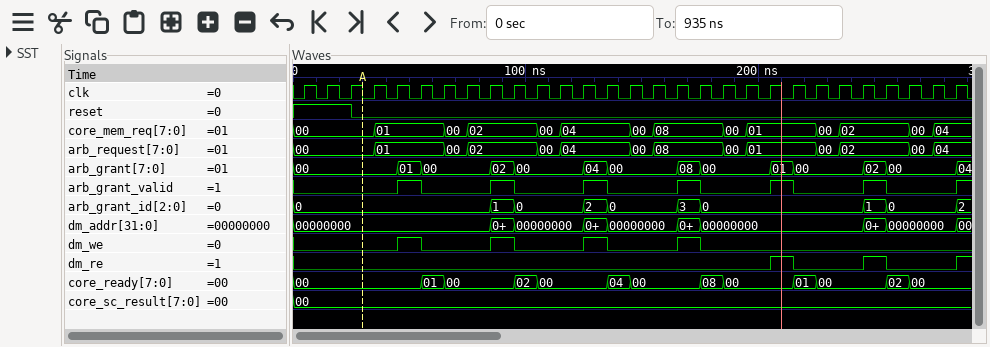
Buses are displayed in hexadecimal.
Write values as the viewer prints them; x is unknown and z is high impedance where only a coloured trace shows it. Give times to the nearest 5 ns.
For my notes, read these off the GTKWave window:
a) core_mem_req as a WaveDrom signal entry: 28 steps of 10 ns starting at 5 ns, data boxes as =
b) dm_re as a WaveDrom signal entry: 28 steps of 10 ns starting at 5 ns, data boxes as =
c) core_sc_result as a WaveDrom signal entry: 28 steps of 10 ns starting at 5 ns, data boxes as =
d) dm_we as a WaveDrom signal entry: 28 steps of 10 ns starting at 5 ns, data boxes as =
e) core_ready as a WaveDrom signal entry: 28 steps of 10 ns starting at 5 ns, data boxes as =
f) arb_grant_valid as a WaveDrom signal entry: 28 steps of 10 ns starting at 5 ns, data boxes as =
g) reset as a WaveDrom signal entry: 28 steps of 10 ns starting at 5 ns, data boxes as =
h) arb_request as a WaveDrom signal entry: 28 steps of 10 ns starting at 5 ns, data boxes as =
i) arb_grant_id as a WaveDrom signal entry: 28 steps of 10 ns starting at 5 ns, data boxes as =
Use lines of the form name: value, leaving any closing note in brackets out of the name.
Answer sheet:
core_mem_req as a WaveDrom signal entry: 28 steps of 10 ns starting at 5 ns, data boxes as =: {name: 'core_mem_req', wave: '=..=..==..==..==..==..==..==', data: '00 01 00 02 00 04 00 08 00 01 00 02 00 04'}
dm_re as a WaveDrom signal entry: 28 steps of 10 ns starting at 5 ns, data boxes as =: {name: 'dm_re', wave: '0...................10..10..'}
core_sc_result as a WaveDrom signal entry: 28 steps of 10 ns starting at 5 ns, data boxes as =: {name: 'core_sc_result', wave: '=...........................', data: '00'}
dm_we as a WaveDrom signal entry: 28 steps of 10 ns starting at 5 ns, data boxes as =: {name: 'dm_we', wave: '0...10..10..10..10..........'}
core_ready as a WaveDrom signal entry: 28 steps of 10 ns starting at 5 ns, data boxes as =: {name: 'core_ready', wave: '=....==..==..==..==..==..==.', data: '00 01 00 02 00 04 00 08 00 01 00 02 00'}
arb_grant_valid as a WaveDrom signal entry: 28 steps of 10 ns starting at 5 ns, data boxes as =: {name: 'arb_grant_valid', wave: '0...10..10..10..10..10..10..'}
reset as a WaveDrom signal entry: 28 steps of 10 ns starting at 5 ns, data boxes as =: {name: 'reset', wave: '1.0.........................'}
arb_request as a WaveDrom signal entry: 28 steps of 10 ns starting at 5 ns, data boxes as =: {name: 'arb_request', wave: '=..=..==..==..==..==..==..==', data: '00 01 00 02 00 04 00 08 00 01 00 02 00 04'}
arb_grant_id as a WaveDrom signal entry: 28 steps of 10 ns starting at 5 ns, data boxes as =: {name: 'arb_grant_id', wave: '=.......==..==..==......==..', data: '0 1 0 2 0 3 0 1 0'}
